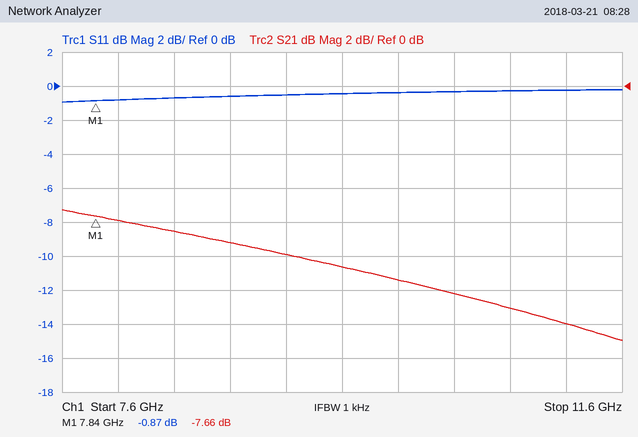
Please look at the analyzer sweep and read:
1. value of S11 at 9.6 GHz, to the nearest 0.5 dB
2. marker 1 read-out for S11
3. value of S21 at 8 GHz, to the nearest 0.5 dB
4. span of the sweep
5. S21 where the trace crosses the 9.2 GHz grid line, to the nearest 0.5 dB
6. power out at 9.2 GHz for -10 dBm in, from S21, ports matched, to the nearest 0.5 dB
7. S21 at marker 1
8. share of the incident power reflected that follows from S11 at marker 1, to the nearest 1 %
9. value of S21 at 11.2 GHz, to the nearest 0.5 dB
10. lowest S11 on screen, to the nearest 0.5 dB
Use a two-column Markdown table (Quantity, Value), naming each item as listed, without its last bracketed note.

| Quantity | Value |
|---|---|
| value of S11 at 9.6 GHz, to the nearest 0.5 dB | -0.5 dB |
| marker 1 read-out for S11 | -0.87 dB |
| value of S21 at 8 GHz, to the nearest 0.5 dB | -8.0 dB |
| span of the sweep | 4 GHz |
| S21 where the trace crosses the 9.2 GHz grid line, to the nearest 0.5 dB | -10.0 dB |
| power out at 9.2 GHz for -10 dBm in, from S21, ports matched, to the nearest 0.5 dB | -20.0 dBm |
| S21 at marker 1 | -7.66 dB |
| share of the incident power reflected that follows from S11 at marker 1, to the nearest 1 % | 82 % |
| value of S21 at 11.2 GHz, to the nearest 0.5 dB | -14.0 dB |
| lowest S11 on screen, to the nearest 0.5 dB | -1.0 dB |
